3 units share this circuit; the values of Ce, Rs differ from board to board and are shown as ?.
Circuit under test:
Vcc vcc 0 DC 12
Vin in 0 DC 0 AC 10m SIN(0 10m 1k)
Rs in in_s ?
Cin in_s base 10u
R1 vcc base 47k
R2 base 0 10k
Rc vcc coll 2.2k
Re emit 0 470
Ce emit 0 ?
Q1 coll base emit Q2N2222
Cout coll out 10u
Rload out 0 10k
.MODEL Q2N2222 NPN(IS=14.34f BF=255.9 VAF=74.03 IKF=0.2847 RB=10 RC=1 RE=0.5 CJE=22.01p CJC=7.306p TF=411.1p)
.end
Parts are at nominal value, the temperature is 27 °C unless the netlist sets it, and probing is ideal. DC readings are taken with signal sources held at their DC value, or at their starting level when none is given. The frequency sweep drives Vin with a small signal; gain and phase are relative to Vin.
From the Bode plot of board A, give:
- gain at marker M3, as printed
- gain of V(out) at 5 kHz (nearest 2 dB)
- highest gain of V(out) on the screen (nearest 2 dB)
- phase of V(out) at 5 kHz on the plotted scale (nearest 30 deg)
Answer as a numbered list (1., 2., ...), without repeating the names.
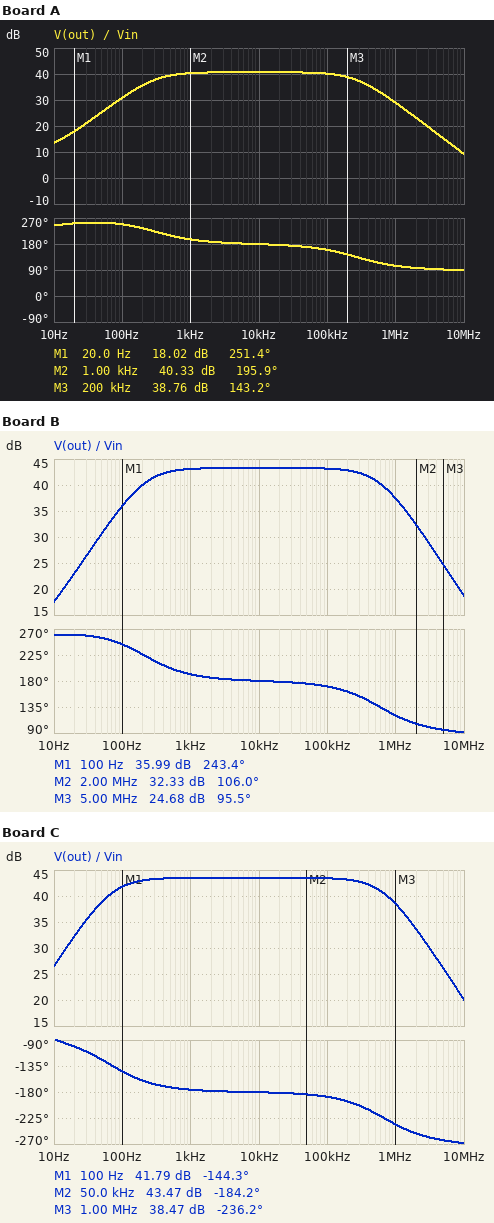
1. 38.76 dB
2. 40 dB
3. 40 dB
4. 180 deg
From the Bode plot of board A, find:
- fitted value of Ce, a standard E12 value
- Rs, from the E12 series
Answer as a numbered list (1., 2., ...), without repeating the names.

1. 39 µF
2. 1.2 kΩ
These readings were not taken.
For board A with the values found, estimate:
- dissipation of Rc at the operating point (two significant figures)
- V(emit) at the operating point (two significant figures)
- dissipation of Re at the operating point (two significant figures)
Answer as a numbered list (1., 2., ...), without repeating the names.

1. 18 mW
2. 1.3 V
3. 3.8 mW
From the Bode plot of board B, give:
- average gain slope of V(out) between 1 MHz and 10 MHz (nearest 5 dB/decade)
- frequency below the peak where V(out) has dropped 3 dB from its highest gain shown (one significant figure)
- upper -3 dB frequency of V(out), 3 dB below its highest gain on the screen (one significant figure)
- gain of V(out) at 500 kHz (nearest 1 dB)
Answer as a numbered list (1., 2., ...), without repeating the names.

1. -20 dB/decade
2. 200 Hz
3. 600 kHz
4. 41 dB
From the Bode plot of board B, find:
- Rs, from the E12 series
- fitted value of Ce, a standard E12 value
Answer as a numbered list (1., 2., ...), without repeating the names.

1. 390 Ω
2. 68 µF
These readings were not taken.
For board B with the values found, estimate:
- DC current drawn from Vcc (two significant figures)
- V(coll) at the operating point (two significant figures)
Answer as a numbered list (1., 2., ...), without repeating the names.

1. 3.1 mA
2. 5.7 V
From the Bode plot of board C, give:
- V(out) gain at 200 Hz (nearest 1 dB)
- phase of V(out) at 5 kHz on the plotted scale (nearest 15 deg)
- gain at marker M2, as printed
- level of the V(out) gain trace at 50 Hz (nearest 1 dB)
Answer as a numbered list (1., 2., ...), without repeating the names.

1. 43 dB
2. -180 deg
3. 43.47 dB
4. 39 dB
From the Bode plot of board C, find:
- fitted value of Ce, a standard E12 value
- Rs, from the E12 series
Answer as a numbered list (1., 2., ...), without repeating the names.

1. 220 µF
2. 330 Ω
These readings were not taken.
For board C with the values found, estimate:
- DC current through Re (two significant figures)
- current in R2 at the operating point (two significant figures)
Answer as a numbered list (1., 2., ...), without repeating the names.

1. 2.9 mA
2. 200 µA
